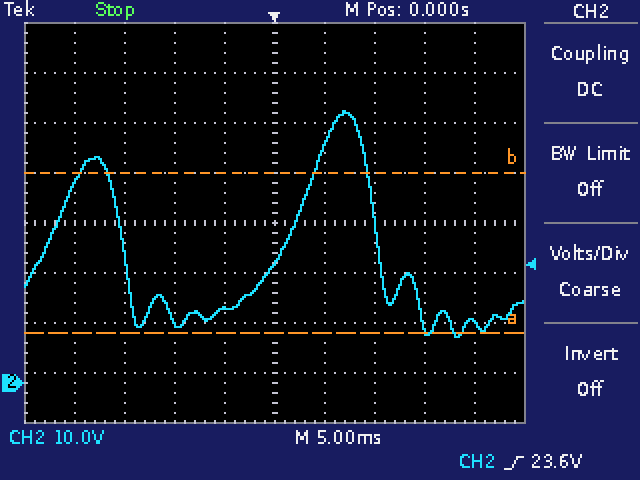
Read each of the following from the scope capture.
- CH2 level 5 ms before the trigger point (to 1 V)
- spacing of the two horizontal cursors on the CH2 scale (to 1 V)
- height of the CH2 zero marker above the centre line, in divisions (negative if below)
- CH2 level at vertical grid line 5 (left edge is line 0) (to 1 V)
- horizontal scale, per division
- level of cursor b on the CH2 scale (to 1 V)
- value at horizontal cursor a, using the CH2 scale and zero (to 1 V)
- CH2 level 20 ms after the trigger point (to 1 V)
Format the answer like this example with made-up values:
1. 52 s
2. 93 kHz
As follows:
1. 15 V
2. 32 V
3. -3.2 div
4. 24 V
5. 5 ms
6. 42 V
7. 10 V
8. 12 V
